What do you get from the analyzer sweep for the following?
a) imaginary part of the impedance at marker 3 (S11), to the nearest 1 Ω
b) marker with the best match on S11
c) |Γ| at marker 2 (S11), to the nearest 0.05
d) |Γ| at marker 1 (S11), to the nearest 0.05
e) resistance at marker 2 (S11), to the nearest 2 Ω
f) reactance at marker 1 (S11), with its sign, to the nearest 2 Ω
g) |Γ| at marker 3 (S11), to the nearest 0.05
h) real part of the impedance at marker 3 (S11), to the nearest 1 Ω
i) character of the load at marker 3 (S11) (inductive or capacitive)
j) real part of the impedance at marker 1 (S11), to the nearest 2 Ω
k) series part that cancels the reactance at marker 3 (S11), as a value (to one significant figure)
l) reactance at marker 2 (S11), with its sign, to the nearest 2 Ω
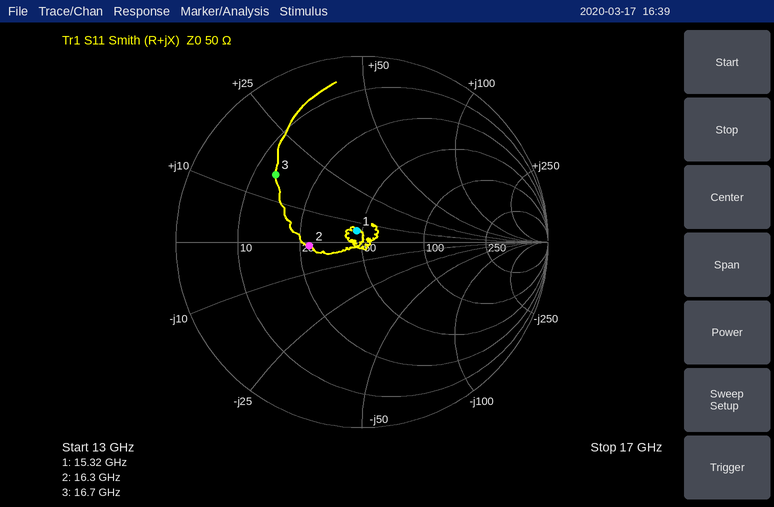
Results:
+16 Ω
marker 1
0.30
0.05
28 Ω
+6 Ω
0.60
14 Ω
inductive
46 Ω
600 fF
-2 Ω
